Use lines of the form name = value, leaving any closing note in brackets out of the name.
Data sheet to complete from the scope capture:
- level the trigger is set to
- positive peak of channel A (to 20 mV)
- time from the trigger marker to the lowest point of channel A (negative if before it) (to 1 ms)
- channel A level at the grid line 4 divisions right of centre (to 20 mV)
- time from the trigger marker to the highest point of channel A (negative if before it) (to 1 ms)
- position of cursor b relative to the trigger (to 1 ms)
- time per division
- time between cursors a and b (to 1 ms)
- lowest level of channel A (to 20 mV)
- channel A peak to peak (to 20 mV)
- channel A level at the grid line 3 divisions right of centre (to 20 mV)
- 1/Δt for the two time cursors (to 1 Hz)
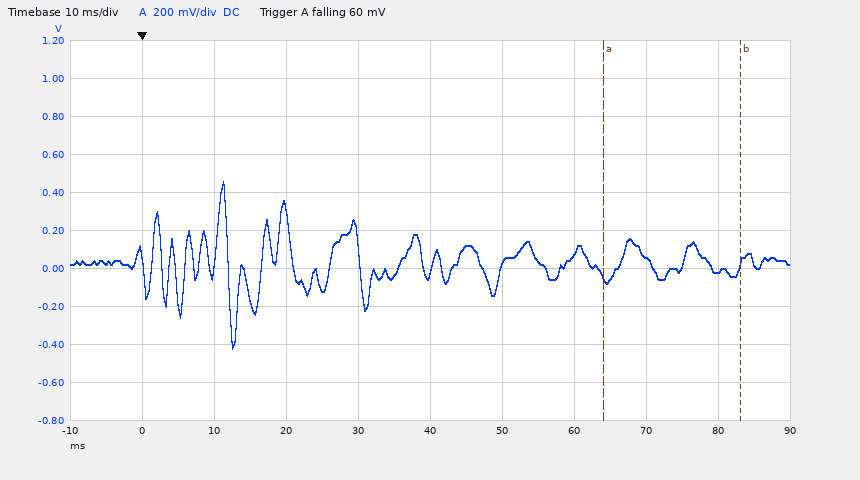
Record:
level the trigger is set to = 60 mV
positive peak of channel A = 460 mV
time from the trigger marker to the lowest point of channel A (negative if before it) = +13 ms
channel A level at the grid line 4 divisions right of centre = -20 mV
time from the trigger marker to the highest point of channel A (negative if before it) = +11 ms
position of cursor b relative to the trigger = +83 ms
time per division = 10 ms
time between cursors a and b = 19 ms
lowest level of channel A = -420 mV
channel A peak to peak = 880 mV
channel A level at the grid line 3 divisions right of centre = 60 mV
1/Δt for the two time cursors = 53 Hz
